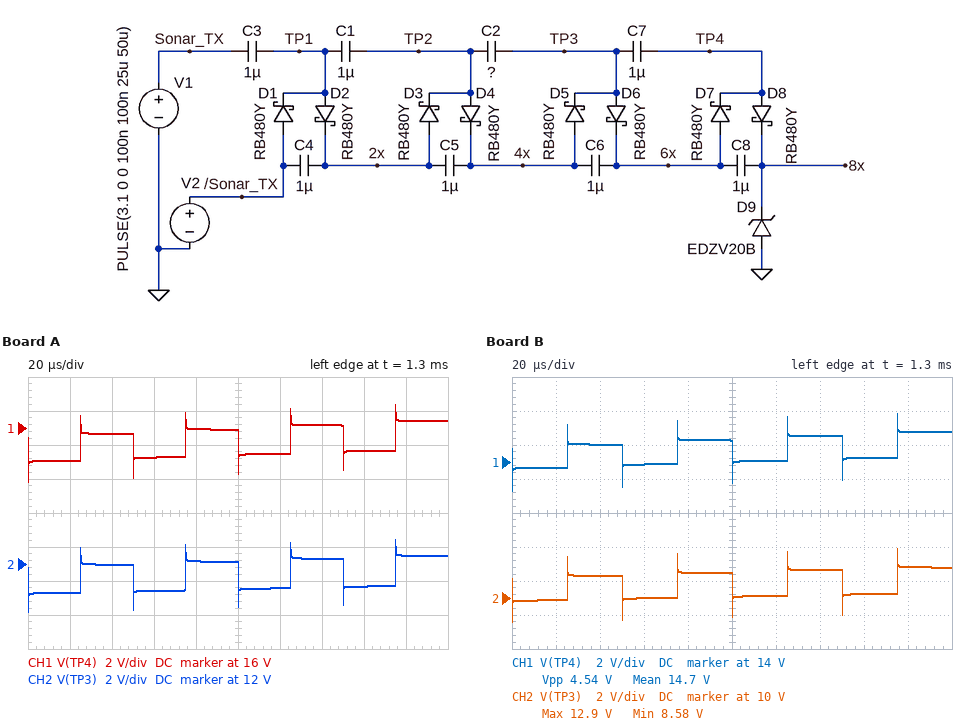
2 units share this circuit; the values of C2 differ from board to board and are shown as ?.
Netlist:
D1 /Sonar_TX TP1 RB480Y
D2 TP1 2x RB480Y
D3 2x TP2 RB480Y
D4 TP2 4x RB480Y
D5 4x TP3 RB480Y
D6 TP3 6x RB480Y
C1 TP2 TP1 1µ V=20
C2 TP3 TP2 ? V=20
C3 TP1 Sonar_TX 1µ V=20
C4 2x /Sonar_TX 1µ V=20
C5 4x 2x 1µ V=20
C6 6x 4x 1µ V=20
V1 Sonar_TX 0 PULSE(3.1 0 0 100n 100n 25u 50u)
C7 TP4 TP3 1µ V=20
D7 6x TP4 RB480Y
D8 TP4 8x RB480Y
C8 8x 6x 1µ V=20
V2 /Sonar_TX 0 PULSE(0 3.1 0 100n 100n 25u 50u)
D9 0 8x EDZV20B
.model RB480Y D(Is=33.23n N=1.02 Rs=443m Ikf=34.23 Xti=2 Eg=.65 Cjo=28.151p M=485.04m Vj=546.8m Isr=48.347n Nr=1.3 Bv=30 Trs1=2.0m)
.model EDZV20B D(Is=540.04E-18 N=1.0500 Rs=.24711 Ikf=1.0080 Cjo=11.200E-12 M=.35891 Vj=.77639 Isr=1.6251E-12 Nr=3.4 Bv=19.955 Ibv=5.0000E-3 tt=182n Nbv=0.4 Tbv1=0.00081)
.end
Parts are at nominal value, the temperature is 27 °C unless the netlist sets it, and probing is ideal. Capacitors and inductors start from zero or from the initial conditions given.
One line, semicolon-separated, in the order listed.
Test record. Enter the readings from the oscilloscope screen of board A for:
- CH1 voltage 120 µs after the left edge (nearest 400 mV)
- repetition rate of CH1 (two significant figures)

14.4 V; 20 kHz
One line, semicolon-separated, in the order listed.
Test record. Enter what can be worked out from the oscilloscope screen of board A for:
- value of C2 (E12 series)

3.9 µF
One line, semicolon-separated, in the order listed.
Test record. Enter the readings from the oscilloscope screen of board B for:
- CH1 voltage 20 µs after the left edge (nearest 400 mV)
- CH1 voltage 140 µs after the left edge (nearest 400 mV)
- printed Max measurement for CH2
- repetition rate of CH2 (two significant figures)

13.6 V; 15.6 V; 12.9 V; 20 kHz
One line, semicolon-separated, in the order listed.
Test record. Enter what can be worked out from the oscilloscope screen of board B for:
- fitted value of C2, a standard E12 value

5.6 µF
